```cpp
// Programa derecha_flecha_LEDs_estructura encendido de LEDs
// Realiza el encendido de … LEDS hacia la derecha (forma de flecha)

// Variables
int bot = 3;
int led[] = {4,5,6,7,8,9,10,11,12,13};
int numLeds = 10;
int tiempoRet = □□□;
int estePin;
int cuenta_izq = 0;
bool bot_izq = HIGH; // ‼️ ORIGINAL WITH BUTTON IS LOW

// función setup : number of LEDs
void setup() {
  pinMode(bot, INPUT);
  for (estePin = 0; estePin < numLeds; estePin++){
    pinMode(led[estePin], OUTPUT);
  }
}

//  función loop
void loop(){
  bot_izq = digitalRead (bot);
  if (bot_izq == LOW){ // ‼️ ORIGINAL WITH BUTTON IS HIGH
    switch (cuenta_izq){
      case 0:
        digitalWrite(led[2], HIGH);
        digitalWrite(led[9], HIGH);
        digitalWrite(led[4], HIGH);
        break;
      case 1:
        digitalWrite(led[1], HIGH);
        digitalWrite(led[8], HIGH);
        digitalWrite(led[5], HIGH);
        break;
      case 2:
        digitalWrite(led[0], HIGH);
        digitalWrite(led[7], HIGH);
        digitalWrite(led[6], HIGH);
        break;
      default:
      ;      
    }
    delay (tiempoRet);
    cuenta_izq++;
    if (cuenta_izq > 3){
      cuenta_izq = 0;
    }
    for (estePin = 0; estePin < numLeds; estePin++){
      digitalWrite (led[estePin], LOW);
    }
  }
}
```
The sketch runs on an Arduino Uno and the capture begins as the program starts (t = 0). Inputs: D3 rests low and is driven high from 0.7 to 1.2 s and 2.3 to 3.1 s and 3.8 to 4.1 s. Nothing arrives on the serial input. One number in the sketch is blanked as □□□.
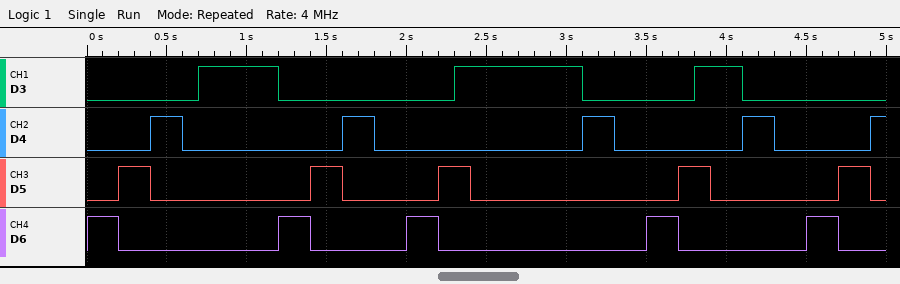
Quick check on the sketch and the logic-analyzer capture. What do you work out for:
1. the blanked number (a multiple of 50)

200
